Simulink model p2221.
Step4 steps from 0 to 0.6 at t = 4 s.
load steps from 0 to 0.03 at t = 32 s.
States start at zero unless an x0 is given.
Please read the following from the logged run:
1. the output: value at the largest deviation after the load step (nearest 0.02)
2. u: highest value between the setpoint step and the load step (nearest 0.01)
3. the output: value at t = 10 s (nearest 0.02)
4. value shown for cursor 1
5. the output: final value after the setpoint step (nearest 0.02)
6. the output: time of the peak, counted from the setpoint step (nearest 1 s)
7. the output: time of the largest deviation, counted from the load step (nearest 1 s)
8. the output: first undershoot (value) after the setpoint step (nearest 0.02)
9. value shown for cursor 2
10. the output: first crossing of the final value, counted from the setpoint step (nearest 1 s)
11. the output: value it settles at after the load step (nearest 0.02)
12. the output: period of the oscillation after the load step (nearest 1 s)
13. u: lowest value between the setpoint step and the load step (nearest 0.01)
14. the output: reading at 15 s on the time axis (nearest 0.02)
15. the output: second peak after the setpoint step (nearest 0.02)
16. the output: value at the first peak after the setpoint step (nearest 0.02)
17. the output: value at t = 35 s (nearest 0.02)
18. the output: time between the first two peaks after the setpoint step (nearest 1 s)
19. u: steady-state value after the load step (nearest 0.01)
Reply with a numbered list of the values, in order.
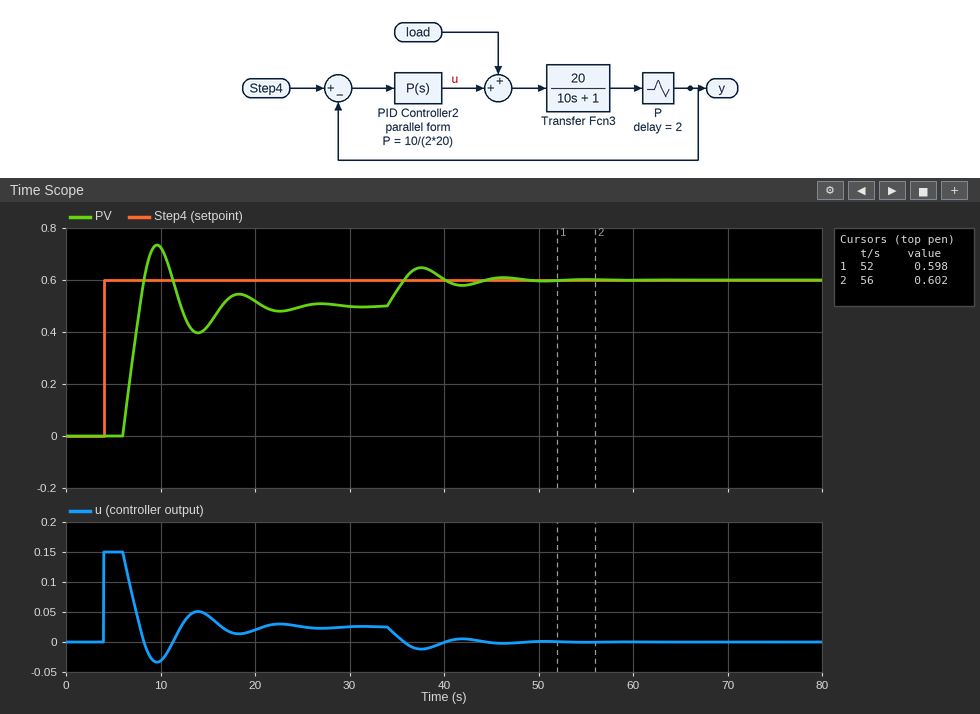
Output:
1. 0.64
2. 0.15
3. 0.72
4. 0.598
5. 0.50
6. 6 s
7. 6 s
8. 0.40
9. 0.602
10. 4 s
11. 0.60
12. 9 s
13. -0.03
14. 0.42
15. 0.54
16. 0.74
17. 0.56
18. 9 s
19. 0.00
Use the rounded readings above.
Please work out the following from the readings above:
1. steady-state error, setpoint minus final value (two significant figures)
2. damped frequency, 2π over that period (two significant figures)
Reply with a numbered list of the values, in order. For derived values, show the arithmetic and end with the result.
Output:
1. 0.6 - 0.5 = 0.10
2. 2π / 9 = 0.70 rad/s
